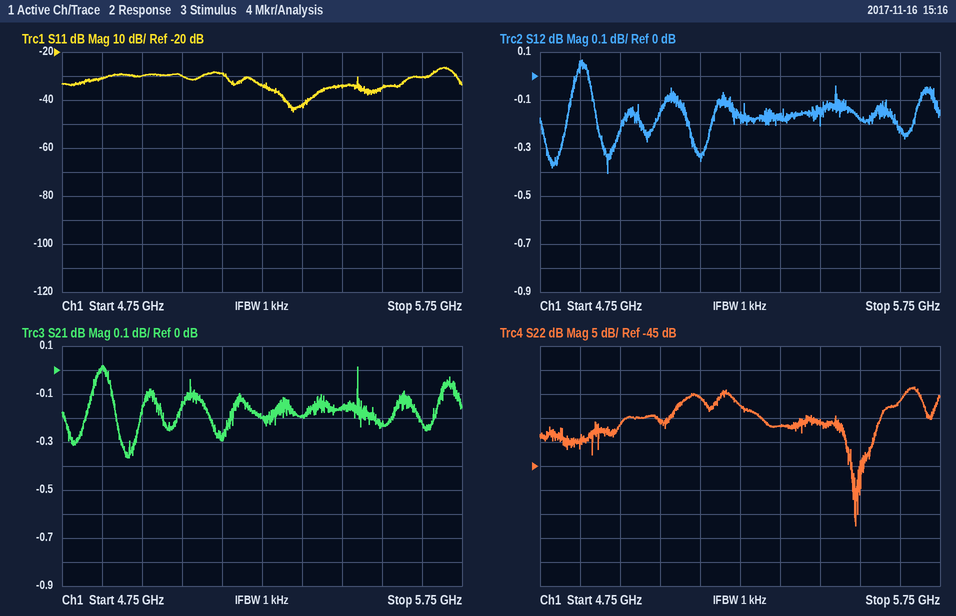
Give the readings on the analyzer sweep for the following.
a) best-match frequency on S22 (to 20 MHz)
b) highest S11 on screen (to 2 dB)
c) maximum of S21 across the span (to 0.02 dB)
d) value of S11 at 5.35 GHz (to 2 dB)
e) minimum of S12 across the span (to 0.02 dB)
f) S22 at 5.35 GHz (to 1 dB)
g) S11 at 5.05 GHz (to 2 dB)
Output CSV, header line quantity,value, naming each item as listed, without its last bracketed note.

quantity,value
best-match frequency on S22,5.54 GHz
highest S11 on screen,-26 dB
maximum of S21 across the span,0.02 dB
value of S11 at 5.35 GHz,-42 dB
minimum of S12 across the span,-0.40 dB
S22 at 5.35 GHz,-37 dB
S11 at 5.05 GHz,-30 dB
